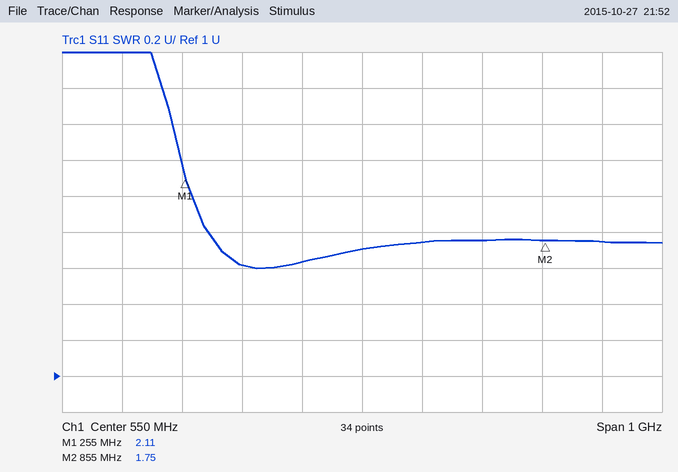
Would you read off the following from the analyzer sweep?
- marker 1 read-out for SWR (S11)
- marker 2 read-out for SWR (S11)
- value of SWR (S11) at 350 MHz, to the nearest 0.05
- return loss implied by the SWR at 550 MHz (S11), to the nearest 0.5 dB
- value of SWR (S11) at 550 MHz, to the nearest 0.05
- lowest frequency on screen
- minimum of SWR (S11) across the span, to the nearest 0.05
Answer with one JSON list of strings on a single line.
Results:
["2.11", "1.75", "1.60", "11.5 dB", "1.70", "50 MHz", "1.60"]
